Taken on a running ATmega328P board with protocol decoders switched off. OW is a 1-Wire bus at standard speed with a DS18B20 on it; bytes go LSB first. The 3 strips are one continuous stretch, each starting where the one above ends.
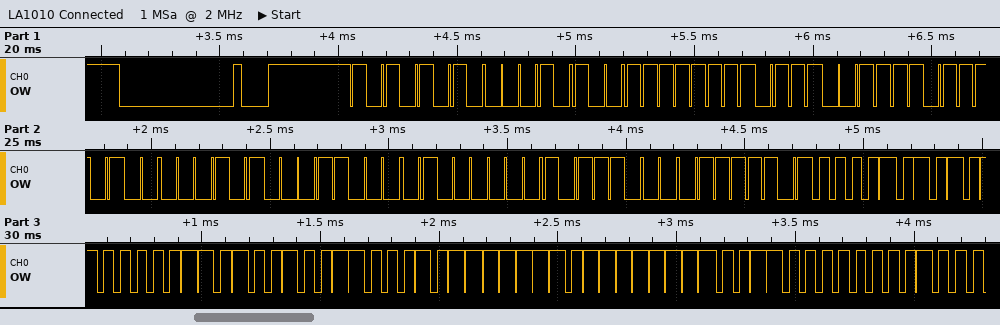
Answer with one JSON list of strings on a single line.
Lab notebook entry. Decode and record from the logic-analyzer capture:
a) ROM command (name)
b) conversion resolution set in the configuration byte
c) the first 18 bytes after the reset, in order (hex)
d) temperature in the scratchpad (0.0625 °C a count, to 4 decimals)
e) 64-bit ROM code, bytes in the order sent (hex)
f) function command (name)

["Match ROM", "12 bits", "55 28 FF CE BB A0 18 02 1D BE 50 05 4B 46 7F FF 0C 10", "85.0000 °C", "28 FF CE BB A0 18 02 1D", "Read Scratchpad"]
